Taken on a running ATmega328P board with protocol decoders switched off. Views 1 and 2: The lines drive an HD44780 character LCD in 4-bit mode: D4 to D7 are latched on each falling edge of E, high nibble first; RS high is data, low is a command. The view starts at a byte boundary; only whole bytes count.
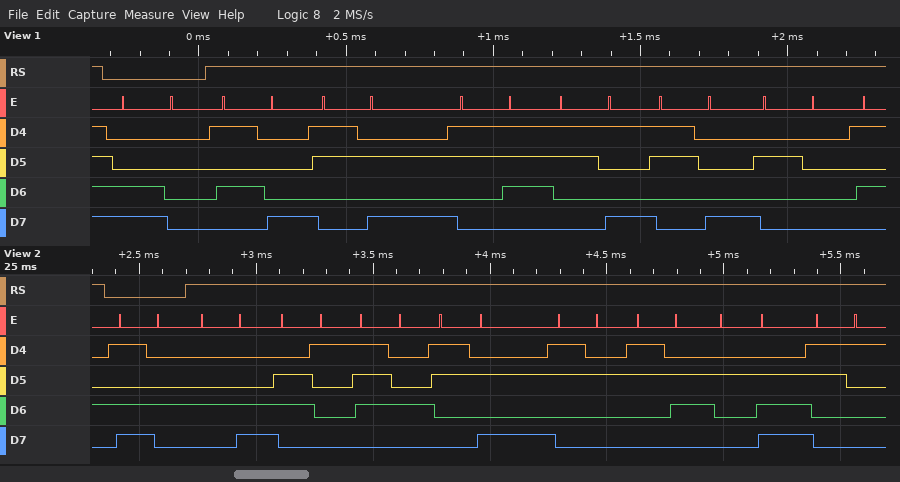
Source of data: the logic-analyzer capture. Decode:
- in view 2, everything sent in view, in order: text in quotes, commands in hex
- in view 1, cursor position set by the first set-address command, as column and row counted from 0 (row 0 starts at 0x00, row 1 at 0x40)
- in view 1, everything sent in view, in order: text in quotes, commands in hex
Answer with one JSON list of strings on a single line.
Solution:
["0xD4 \"Lat:26.1\"", "column 0, row 1", "0xC0 \"X:798 \""]
